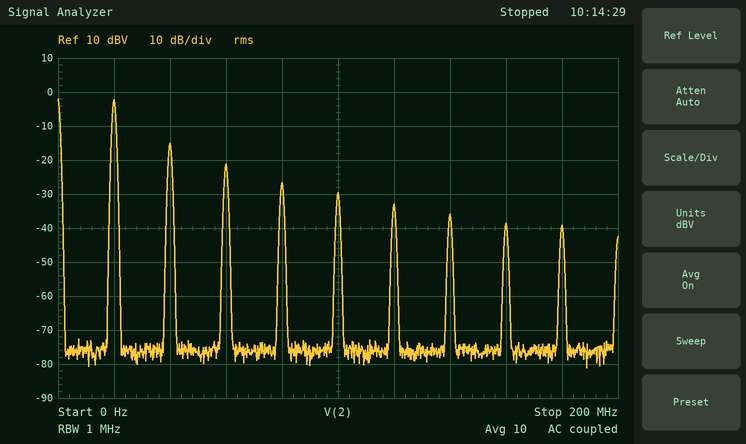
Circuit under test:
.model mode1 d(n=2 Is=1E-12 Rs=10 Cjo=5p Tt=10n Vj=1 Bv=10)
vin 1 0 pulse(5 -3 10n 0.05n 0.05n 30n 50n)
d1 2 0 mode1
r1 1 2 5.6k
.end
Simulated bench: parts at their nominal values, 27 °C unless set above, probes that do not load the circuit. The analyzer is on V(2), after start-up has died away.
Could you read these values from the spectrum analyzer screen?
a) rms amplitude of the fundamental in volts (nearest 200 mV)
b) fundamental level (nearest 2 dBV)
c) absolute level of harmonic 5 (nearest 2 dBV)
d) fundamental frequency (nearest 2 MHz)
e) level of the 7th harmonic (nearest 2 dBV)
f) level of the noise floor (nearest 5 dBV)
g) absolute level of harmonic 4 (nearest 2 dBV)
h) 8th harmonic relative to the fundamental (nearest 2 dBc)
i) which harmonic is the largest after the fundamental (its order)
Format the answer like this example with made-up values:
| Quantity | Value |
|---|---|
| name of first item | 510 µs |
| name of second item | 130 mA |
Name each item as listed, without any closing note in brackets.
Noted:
| Quantity | Value |
|---|---|
| rms amplitude of the fundamental in volts | 800 mV |
| fundamental level | -2 dBV |
| absolute level of harmonic 5 | -30 dBV |
| fundamental frequency | 20 MHz |
| level of the 7th harmonic | -36 dBV |
| level of the noise floor | -75 dBV |
| absolute level of harmonic 4 | -26 dBV |
| 8th harmonic relative to the fundamental | -36 dBc |
| which harmonic is the largest after the fundamental | 2 |
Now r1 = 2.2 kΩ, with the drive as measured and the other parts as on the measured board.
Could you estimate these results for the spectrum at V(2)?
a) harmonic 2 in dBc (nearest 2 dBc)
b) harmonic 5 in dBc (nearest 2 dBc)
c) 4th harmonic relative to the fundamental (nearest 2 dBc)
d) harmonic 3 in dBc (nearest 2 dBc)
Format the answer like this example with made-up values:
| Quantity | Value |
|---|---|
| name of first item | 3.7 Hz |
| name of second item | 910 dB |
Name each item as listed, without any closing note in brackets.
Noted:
| Quantity | Value |
|---|---|
| harmonic 2 in dBc | -12 dBc |
| harmonic 5 in dBc | -24 dBc |
| 4th harmonic relative to the fundamental | -20 dBc |
| harmonic 3 in dBc | -16 dBc |
